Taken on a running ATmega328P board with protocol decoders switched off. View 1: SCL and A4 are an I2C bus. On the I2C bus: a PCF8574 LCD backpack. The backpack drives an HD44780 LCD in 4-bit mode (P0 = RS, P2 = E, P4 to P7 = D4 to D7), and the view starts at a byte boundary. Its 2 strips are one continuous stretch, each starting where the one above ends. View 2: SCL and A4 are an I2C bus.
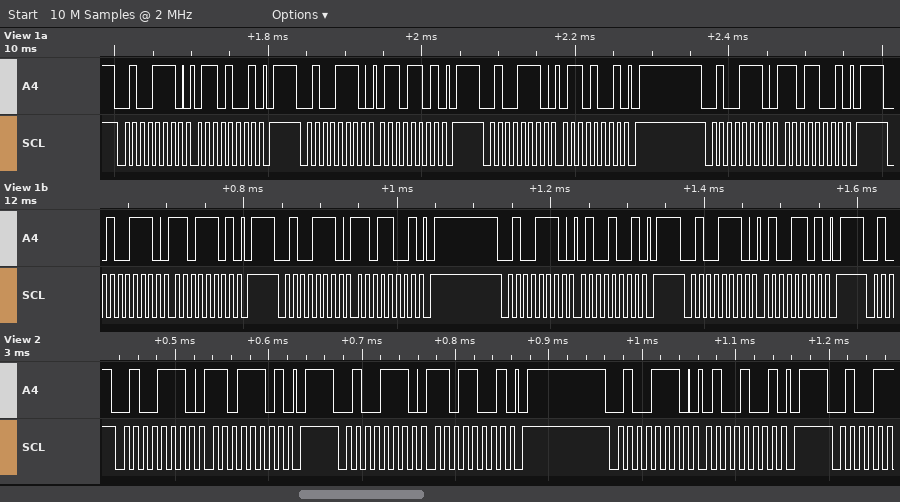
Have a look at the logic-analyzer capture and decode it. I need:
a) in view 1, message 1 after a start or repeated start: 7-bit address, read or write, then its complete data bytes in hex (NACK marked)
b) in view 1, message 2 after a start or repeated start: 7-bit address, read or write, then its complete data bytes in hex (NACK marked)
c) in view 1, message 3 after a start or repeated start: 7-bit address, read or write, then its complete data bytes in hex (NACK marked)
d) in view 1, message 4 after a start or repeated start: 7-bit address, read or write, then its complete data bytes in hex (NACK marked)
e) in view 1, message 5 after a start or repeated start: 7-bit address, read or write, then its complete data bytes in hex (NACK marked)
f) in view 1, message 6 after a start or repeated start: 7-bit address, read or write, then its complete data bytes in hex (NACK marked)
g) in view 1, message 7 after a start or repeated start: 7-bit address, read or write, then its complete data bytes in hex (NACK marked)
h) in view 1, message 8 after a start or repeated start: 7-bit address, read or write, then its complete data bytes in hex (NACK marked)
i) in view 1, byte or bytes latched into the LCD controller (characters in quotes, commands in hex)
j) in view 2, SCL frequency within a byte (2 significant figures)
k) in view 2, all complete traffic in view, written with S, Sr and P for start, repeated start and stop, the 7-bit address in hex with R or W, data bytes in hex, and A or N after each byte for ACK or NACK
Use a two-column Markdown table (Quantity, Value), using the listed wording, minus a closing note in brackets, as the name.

| Quantity | Value |
|---|---|
| in view 1, message 1 after a start or repeated start: 7-bit address, read or write, then its complete data bytes in hex | 0x27 write: 69 |
| in view 1, message 2 after a start or repeated start: 7-bit address, read or write, then its complete data bytes in hex | 0x27 write: 6D |
| in view 1, message 3 after a start or repeated start: 7-bit address, read or write, then its complete data bytes in hex | 0x27 write: 69 |
| in view 1, message 4 after a start or repeated start: 7-bit address, read or write, then its complete data bytes in hex | 0x27 write: D9 |
| in view 1, message 5 after a start or repeated start: 7-bit address, read or write, then its complete data bytes in hex | 0x27 write: DD |
| in view 1, message 6 after a start or repeated start: 7-bit address, read or write, then its complete data bytes in hex | 0x27 write: D9 |
| in view 1, message 7 after a start or repeated start: 7-bit address, read or write, then its complete data bytes in hex | 0x27 write: 49 |
| in view 1, message 8 after a start or repeated start: 7-bit address, read or write, then its complete data bytes in hex | 0x27 write: 4D |
| in view 1, byte or bytes latched into the LCD controller | 'm' |
| in view 2, SCL frequency within a byte | 100 kHz |
| in view 2, all complete traffic in view, written with S, Sr and P for start, repeated start and stop, the 7-bit address in hex with R or W, data bytes in hex, and A or N after each byte for ACK or NACK | S 27W A DD A P S 27W A D9 A P S 27W A 49 A P |
